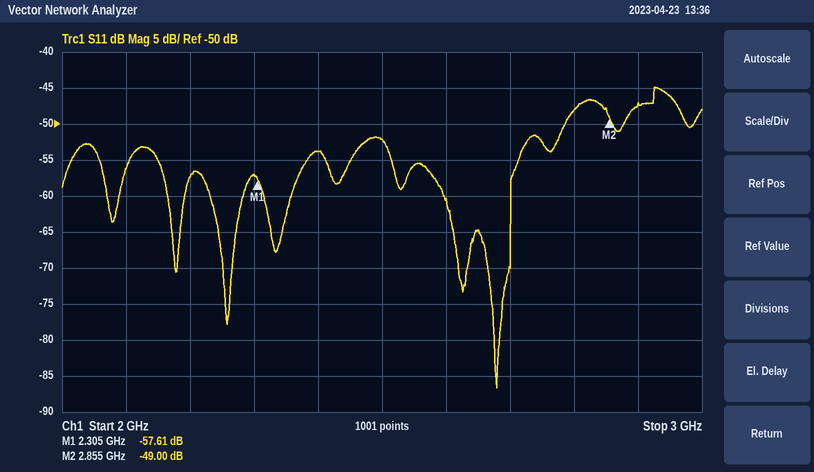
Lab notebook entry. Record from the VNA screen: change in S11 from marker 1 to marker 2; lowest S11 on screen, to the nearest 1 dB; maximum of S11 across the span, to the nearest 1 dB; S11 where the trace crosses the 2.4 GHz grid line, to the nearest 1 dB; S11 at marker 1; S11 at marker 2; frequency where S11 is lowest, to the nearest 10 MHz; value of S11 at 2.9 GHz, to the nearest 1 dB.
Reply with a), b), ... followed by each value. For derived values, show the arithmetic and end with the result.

a) -49 − (-57.61) = 8.61 dB
b) -87 dB
c) -45 dB
d) -54 dB
e) -57.61 dB
f) -49.00 dB
g) 2.68 GHz
h) -47 dB
